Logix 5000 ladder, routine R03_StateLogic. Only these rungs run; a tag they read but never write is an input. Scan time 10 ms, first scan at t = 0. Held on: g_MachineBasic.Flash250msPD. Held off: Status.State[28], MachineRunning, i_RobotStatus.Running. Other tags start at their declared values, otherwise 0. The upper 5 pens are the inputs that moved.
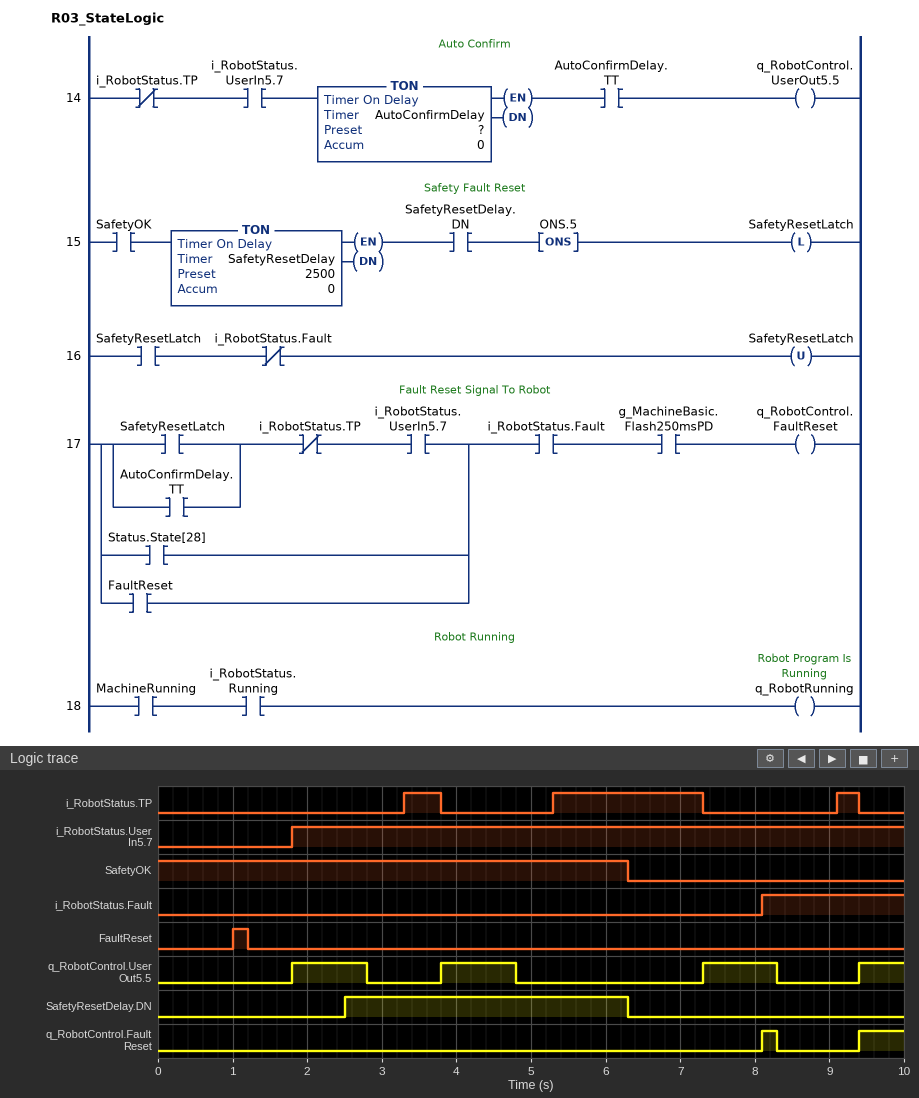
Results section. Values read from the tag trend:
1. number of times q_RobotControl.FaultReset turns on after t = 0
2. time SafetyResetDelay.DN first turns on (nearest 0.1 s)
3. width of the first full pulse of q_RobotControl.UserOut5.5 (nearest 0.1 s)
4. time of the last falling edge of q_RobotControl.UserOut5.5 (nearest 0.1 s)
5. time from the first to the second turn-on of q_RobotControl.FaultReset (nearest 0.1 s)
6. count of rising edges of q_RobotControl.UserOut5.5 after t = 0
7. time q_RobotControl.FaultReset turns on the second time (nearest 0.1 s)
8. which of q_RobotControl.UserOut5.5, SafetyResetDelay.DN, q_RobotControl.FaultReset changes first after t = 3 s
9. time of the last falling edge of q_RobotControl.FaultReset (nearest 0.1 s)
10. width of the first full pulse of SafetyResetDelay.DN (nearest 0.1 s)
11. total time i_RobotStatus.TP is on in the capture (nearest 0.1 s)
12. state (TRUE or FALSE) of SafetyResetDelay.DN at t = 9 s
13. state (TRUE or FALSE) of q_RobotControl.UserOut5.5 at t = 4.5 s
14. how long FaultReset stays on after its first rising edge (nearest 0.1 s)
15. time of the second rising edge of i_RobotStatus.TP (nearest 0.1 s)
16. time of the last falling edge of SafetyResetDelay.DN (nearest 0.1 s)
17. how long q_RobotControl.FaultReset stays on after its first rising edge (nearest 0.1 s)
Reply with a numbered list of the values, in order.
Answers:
1. 2
2. 2.5 s
3. 1.0 s
4. 8.3 s
5. 1.3 s
6. 4
7. 9.4 s
8. q_RobotControl.UserOut5.5
9. 8.3 s
10. 3.8 s
11. 2.8 s
12. FALSE
13. TRUE
14. 0.2 s
15. 5.3 s
16. 6.3 s
17. 0.2 s
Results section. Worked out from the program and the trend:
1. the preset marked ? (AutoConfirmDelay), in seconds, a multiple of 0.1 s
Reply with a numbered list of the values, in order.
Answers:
1. 1.0 s
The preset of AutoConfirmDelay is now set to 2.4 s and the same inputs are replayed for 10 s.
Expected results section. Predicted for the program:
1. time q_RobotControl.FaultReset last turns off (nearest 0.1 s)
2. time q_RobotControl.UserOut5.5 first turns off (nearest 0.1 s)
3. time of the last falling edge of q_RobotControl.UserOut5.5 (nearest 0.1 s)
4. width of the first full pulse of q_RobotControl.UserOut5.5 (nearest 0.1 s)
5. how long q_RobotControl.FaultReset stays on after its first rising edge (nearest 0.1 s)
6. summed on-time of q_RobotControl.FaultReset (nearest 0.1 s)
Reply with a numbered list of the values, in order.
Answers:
1. 9.1 s
2. 3.3 s
3. 9.1 s
4. 1.5 s
5. 1.0 s
6. 1.6 s
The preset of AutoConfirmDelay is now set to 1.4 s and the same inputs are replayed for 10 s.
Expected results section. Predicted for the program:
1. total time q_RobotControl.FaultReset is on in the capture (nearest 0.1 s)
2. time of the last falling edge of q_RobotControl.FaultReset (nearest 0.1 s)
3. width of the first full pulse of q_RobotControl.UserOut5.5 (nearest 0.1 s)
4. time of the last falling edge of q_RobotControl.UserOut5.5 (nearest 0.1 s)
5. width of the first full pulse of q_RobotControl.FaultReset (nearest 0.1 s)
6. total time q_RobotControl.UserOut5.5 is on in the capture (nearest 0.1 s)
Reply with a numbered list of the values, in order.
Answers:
1. 1.2 s
2. 8.7 s
3. 1.4 s
4. 8.7 s
5. 0.6 s
6. 4.8 s
